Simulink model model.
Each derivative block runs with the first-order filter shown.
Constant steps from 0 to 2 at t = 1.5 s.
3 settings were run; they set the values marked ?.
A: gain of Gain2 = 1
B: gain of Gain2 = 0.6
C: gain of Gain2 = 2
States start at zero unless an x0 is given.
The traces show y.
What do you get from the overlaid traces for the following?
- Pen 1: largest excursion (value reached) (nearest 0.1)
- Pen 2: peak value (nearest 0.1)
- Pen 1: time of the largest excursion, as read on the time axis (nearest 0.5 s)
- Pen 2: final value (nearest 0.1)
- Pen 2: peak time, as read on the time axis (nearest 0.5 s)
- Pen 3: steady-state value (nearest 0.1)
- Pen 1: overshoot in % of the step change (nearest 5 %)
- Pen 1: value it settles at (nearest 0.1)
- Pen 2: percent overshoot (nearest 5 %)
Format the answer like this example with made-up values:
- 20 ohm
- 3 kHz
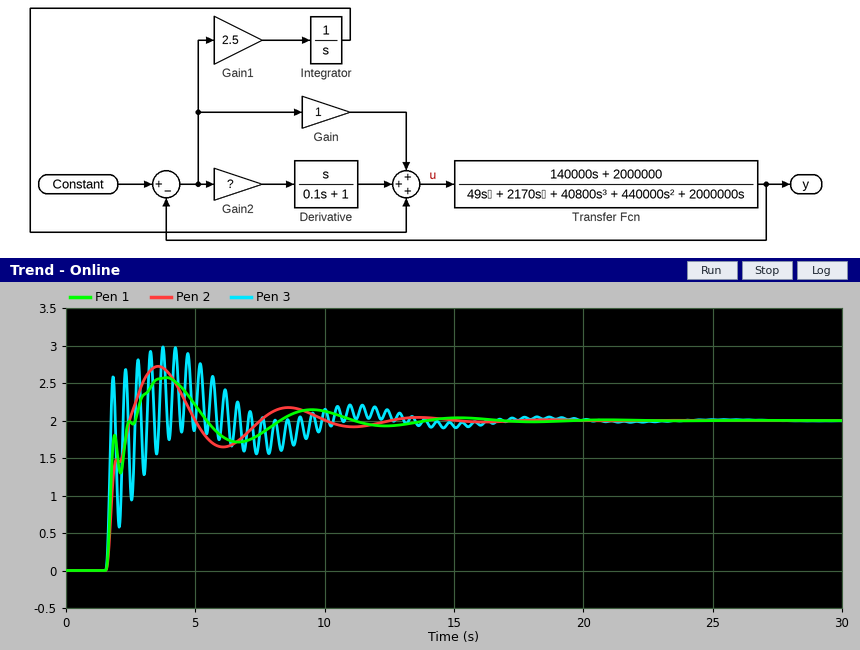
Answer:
- 2.6
- 2.7
- 4.0 s
- 2.0
- 3.5 s
- 2.0
- 30 %
- 2.0
- 35 %
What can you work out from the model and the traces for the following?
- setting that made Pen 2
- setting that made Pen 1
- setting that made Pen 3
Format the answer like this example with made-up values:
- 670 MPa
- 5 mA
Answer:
- B
- A
- C
